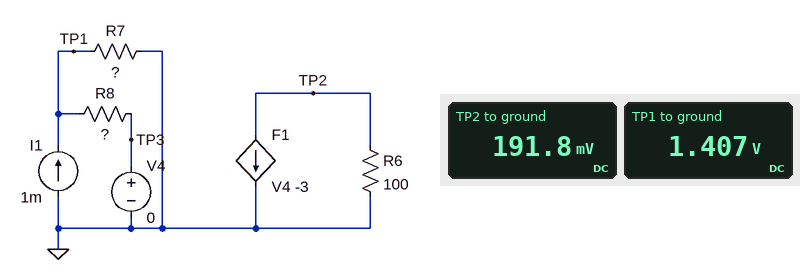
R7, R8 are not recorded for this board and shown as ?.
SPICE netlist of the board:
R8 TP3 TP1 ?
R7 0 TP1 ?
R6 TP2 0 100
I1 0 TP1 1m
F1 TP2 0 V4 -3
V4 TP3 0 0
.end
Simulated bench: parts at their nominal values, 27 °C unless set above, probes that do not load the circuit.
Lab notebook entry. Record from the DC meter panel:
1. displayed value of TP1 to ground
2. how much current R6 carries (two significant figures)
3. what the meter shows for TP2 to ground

1.407 V
1.9 mA
191.8 mV
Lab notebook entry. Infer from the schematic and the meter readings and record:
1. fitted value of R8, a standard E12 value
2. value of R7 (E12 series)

2.2 kΩ
3.9 kΩ
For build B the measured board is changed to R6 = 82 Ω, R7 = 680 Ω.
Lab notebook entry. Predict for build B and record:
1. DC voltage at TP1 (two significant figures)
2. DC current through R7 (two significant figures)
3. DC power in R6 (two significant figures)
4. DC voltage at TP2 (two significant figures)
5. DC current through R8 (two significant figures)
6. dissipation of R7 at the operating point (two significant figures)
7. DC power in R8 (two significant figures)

520 mV
760 µA
41 µW
58 mV
240 µA
400 µW
120 µW
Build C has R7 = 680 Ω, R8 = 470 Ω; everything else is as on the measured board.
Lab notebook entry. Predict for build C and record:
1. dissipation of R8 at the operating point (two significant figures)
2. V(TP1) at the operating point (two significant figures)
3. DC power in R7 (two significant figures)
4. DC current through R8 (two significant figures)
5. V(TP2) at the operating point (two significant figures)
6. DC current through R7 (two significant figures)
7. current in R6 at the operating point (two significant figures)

160 µW
280 mV
110 µW
590 µA
180 mV
410 µA
1.8 mA
